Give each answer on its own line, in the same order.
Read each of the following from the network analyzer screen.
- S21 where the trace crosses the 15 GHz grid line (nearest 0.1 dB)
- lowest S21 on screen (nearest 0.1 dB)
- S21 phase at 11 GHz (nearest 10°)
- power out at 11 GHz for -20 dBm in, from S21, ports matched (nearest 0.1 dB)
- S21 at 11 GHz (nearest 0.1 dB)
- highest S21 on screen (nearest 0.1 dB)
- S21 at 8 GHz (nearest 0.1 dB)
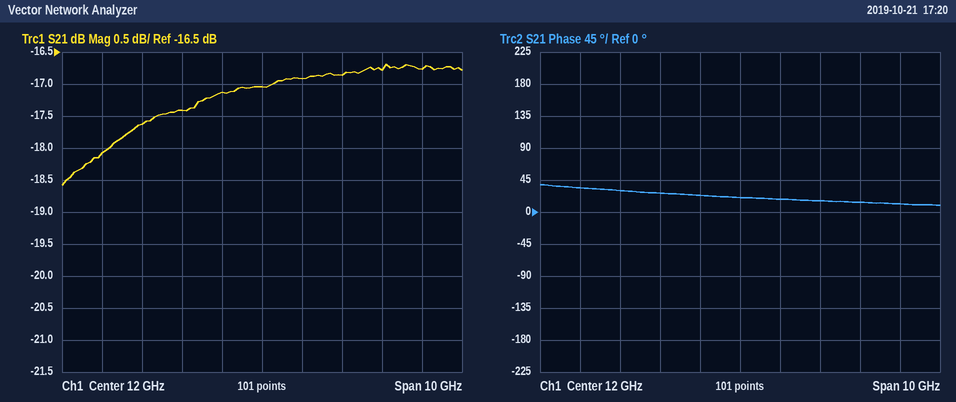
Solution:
-16.8 dB
-18.6 dB
20°
-37.1 dBm
-17.1 dB
-16.7 dB
-18.1 dB
